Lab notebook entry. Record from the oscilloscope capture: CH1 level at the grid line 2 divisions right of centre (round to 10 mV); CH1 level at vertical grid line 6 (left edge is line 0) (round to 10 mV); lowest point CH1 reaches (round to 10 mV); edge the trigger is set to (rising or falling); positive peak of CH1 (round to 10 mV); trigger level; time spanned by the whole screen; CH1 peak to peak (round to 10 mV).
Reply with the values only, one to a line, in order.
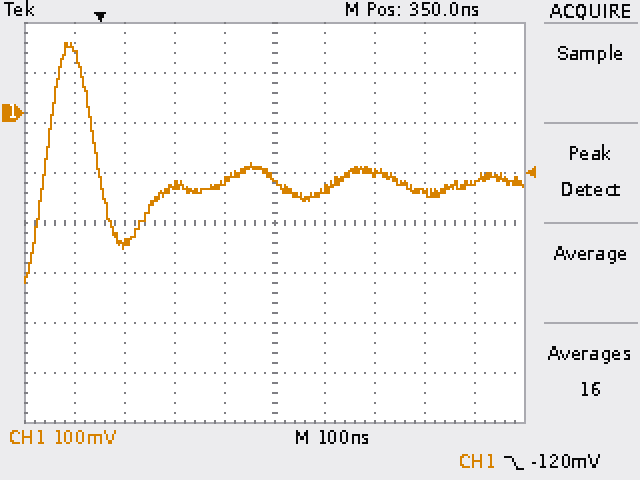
-120 mV
-150 mV
-340 mV
falling
140 mV
-120 mV
1 µs
480 mV
